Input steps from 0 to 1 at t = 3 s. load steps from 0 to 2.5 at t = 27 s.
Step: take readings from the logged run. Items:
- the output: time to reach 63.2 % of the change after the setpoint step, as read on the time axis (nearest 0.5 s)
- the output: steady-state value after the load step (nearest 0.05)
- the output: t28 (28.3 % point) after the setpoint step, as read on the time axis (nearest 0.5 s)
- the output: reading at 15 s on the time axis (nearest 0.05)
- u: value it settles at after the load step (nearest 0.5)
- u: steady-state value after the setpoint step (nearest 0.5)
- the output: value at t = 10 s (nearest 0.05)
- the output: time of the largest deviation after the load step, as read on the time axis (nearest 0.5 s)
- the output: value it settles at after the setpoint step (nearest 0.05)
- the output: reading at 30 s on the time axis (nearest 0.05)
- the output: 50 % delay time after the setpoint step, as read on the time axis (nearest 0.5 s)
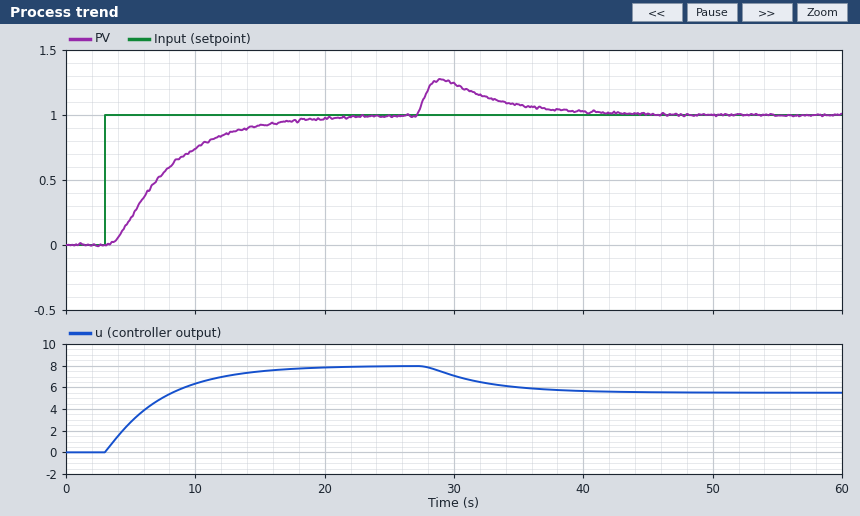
8.5 s
1.00
5.5 s
0.90
5.5
8.0
0.75
29.0 s
1.00
1.25
7.0 s
